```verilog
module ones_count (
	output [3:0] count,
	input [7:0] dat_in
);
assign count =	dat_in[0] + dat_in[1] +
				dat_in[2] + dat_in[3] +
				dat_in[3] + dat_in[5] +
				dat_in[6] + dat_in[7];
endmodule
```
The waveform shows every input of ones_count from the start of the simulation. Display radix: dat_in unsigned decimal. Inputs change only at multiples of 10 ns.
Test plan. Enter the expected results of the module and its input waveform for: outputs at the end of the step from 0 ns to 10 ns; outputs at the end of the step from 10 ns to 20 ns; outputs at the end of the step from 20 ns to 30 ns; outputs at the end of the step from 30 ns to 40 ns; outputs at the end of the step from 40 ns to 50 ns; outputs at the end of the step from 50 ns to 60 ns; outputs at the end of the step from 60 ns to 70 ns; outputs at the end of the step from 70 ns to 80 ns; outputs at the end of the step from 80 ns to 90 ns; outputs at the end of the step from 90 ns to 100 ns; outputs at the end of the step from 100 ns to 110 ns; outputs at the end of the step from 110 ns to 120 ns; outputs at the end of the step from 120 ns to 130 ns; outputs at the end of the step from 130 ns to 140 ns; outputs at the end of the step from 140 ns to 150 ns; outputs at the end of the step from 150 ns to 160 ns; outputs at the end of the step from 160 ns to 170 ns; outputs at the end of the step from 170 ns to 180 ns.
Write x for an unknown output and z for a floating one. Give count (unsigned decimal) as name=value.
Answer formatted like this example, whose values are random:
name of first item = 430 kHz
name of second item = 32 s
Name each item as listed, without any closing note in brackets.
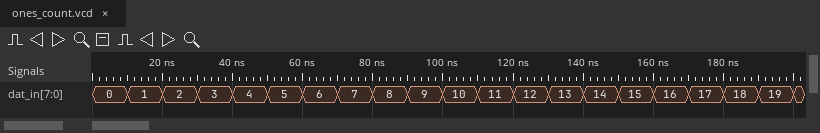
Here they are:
outputs at the end of the step from 0 ns to 10 ns = count=0
outputs at the end of the step from 10 ns to 20 ns = count=1
outputs at the end of the step from 20 ns to 30 ns = count=1
outputs at the end of the step from 30 ns to 40 ns = count=2
outputs at the end of the step from 40 ns to 50 ns = count=1
outputs at the end of the step from 50 ns to 60 ns = count=2
outputs at the end of the step from 60 ns to 70 ns = count=2
outputs at the end of the step from 70 ns to 80 ns = count=3
outputs at the end of the step from 80 ns to 90 ns = count=2
outputs at the end of the step from 90 ns to 100 ns = count=3
outputs at the end of the step from 100 ns to 110 ns = count=3
outputs at the end of the step from 110 ns to 120 ns = count=4
outputs at the end of the step from 120 ns to 130 ns = count=3
outputs at the end of the step from 130 ns to 140 ns = count=4
outputs at the end of the step from 140 ns to 150 ns = count=4
outputs at the end of the step from 150 ns to 160 ns = count=5
outputs at the end of the step from 160 ns to 170 ns = count=0
outputs at the end of the step from 170 ns to 180 ns = count=1
